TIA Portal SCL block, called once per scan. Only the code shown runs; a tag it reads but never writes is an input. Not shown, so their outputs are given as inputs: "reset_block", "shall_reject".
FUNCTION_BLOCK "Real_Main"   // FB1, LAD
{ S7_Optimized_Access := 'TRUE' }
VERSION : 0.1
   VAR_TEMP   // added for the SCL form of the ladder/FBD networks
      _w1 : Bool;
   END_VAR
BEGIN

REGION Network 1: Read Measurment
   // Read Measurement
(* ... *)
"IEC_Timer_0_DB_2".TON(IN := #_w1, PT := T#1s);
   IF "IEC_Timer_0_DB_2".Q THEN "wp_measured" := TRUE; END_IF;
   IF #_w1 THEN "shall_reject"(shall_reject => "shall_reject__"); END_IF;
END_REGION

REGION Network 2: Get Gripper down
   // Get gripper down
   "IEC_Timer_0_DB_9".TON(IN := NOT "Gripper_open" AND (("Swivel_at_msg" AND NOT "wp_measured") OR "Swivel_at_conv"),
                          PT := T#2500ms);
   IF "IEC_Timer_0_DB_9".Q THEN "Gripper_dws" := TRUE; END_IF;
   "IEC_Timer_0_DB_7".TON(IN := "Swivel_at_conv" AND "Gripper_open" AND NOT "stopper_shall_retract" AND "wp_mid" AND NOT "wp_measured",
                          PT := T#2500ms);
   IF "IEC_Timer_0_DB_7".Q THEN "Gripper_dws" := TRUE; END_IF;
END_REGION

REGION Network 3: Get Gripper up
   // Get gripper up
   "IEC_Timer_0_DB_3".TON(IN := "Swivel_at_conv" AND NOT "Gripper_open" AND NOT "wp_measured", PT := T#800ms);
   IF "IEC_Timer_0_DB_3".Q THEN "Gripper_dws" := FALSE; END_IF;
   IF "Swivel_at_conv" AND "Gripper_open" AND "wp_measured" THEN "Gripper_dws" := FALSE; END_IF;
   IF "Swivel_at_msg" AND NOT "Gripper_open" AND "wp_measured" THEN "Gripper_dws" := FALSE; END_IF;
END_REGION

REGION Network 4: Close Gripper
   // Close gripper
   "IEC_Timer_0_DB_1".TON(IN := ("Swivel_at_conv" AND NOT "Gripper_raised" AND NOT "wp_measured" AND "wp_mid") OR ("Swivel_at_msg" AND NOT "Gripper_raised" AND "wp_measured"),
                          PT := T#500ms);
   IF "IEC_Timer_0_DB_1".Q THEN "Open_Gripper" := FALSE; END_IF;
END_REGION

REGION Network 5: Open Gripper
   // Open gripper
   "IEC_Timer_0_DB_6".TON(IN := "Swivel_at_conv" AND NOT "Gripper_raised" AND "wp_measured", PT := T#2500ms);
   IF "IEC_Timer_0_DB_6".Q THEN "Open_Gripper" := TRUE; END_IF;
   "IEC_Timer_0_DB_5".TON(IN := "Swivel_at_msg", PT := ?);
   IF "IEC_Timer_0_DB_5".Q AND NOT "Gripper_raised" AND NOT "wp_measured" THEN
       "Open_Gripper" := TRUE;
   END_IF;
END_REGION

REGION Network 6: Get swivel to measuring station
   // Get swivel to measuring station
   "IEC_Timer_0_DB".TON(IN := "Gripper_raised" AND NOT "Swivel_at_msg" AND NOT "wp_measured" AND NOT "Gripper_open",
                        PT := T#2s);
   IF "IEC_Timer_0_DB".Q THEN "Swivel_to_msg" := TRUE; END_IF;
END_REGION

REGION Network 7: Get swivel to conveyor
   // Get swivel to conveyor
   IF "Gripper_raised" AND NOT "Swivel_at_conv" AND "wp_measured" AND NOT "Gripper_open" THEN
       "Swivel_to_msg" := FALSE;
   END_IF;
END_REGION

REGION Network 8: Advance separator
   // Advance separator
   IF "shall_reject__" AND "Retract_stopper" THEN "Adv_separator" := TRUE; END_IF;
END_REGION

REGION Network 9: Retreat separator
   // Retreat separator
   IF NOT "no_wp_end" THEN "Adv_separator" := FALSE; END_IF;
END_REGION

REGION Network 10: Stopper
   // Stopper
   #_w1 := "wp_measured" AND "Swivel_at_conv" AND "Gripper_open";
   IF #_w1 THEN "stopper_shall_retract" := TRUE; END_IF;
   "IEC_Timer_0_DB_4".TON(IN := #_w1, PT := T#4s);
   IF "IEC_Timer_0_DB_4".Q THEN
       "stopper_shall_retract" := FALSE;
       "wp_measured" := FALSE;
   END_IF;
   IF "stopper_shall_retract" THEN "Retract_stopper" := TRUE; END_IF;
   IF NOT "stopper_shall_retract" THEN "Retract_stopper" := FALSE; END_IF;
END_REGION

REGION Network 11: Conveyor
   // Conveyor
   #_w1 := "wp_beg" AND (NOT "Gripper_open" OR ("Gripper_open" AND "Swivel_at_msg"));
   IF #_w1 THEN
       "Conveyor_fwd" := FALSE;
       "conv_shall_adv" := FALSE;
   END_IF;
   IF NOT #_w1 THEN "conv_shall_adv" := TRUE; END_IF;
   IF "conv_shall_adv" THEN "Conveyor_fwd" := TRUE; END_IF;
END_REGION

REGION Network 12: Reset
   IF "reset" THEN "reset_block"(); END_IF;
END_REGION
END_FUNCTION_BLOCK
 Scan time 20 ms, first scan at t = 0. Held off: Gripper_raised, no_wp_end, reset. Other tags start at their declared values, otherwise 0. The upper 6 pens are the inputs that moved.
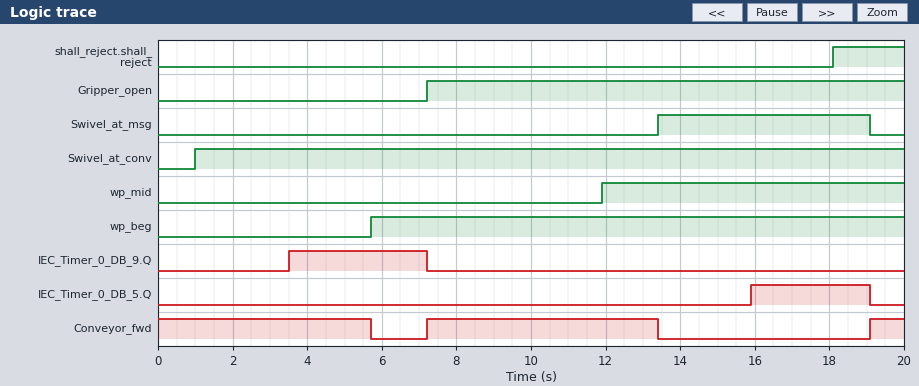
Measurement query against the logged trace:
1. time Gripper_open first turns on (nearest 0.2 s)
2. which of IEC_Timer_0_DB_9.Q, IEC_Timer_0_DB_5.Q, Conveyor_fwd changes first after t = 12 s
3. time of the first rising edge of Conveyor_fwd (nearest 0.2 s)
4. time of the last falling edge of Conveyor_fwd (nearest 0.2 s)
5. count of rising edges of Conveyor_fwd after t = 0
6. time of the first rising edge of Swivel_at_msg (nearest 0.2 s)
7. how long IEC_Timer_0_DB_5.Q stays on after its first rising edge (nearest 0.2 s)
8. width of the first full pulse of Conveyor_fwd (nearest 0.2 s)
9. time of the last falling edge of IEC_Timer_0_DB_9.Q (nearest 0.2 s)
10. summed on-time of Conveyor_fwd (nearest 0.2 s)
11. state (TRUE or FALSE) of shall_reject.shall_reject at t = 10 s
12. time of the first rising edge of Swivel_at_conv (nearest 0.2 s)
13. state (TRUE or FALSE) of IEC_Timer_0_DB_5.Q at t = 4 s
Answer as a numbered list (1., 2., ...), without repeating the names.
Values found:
1. 7.2 s
2. Conveyor_fwd
3. 7.2 s
4. 13.4 s
5. 2
6. 13.4 s
7. 3.2 s
8. 6.2 s
9. 7.2 s
10. 12.8 s
11. FALSE
12. 1.0 s
13. FALSE
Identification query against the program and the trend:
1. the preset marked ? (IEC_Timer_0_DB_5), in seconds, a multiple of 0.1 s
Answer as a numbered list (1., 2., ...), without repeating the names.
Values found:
1. 2.5 s
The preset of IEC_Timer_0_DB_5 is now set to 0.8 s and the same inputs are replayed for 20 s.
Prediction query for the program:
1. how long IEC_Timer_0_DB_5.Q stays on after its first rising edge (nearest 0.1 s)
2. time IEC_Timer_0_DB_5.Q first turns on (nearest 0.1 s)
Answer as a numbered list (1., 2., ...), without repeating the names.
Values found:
1. 4.9 s
2. 14.2 s
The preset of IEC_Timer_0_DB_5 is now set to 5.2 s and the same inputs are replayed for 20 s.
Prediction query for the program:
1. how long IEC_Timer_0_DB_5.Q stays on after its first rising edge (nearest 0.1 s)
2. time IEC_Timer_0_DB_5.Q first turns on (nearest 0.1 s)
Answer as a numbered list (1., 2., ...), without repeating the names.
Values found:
1. 0.5 s
2. 18.6 s
